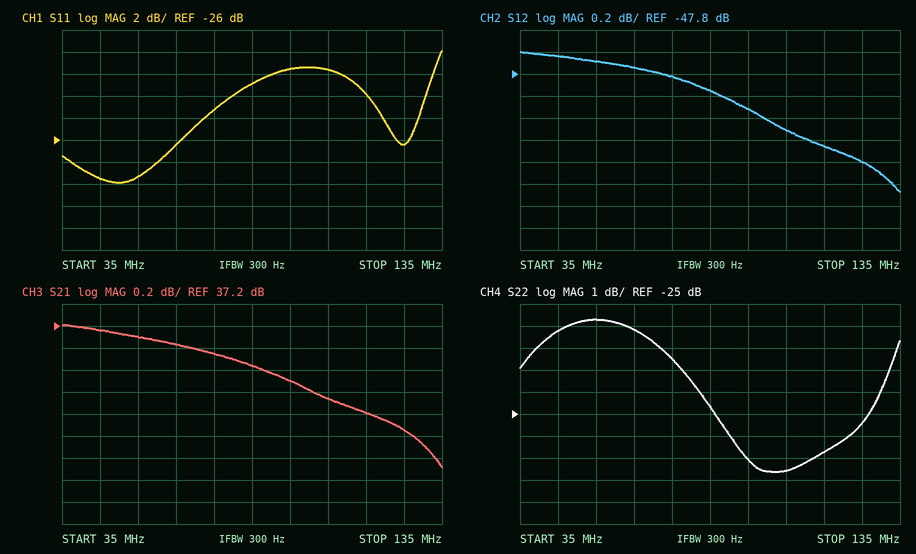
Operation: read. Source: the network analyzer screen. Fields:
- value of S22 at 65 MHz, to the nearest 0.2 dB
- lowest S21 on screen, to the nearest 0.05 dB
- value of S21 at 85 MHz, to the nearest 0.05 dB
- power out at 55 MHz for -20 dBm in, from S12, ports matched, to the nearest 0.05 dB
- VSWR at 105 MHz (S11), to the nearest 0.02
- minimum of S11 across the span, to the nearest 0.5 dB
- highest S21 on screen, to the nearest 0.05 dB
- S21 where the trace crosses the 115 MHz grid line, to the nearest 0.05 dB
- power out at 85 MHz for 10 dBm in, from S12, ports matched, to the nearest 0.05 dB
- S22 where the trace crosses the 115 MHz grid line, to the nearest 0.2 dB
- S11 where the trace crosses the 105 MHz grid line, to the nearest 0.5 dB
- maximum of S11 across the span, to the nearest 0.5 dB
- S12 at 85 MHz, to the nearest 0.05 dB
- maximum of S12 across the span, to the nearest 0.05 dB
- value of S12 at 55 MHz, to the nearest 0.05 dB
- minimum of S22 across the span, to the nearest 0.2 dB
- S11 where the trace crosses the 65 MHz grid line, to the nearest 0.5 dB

-21.2 dB
35.90 dB
36.85 dB
-67.70 dBm
1.24
-30.0 dB
37.20 dB
36.40 dB
-37.95 dBm
-26.8 dB
-19.5 dB
-18.0 dB
-47.95 dB
-47.60 dB
-47.70 dB
-27.6 dB
-26.5 dB
